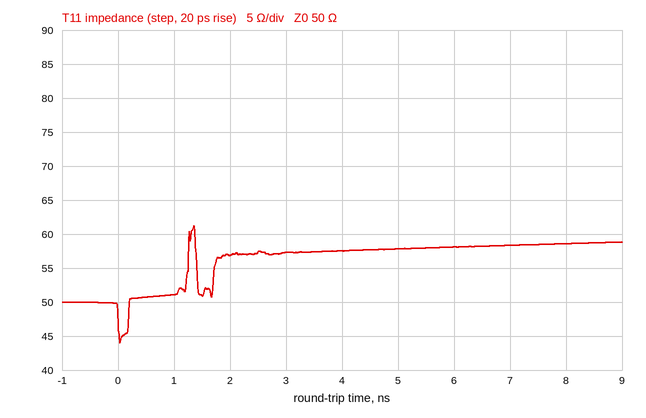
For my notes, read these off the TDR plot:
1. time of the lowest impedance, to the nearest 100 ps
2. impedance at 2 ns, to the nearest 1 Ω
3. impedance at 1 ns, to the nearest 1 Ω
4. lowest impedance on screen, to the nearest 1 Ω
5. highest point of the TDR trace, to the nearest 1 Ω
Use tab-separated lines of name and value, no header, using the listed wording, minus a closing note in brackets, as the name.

time of the lowest impedance, to the nearest 100 ps	0.0 ns
impedance at 2 ns, to the nearest 1 Ω	57 Ω
impedance at 1 ns, to the nearest 1 Ω	51 Ω
lowest impedance on screen, to the nearest 1 Ω	44 Ω
highest point of the TDR trace, to the nearest 1 Ω	61 Ω
